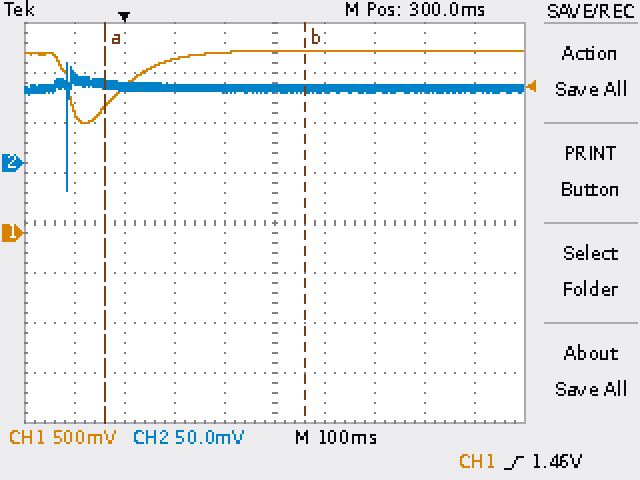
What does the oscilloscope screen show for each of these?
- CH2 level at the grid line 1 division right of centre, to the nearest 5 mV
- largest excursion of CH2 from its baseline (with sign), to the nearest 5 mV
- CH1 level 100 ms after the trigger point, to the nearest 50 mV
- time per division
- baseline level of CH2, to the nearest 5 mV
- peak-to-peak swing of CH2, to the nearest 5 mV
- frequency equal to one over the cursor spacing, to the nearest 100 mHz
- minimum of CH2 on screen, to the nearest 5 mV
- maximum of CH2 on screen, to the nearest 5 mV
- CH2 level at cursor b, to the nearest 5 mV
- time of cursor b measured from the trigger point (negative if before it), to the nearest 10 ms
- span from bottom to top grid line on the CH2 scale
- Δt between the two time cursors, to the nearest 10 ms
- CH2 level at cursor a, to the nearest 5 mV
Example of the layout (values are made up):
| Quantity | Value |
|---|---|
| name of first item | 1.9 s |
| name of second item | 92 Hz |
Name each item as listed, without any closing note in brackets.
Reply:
| Quantity | Value |
|---|---|
| CH2 level at the grid line 1 division right of centre, to the nearest 5 mV | 75 mV |
| largest excursion of CH2 from its baseline (with sign), to the nearest 5 mV | -105 mV |
| CH1 level 100 ms after the trigger point, to the nearest 50 mV | 1.75 V |
| time per division | 100 ms |
| baseline level of CH2, to the nearest 5 mV | 75 mV |
| peak-to-peak swing of CH2, to the nearest 5 mV | 130 mV |
| frequency equal to one over the cursor spacing, to the nearest 100 mHz | 2.5 Hz |
| minimum of CH2 on screen, to the nearest 5 mV | -30 mV |
| maximum of CH2 on screen, to the nearest 5 mV | 100 mV |
| CH2 level at cursor b, to the nearest 5 mV | 75 mV |
| time of cursor b measured from the trigger point (negative if before it), to the nearest 10 ms | +360 ms |
| span from bottom to top grid line on the CH2 scale | 400 mV |
| Δt between the two time cursors, to the nearest 10 ms | 400 ms |
| CH2 level at cursor a, to the nearest 5 mV | 80 mV |
